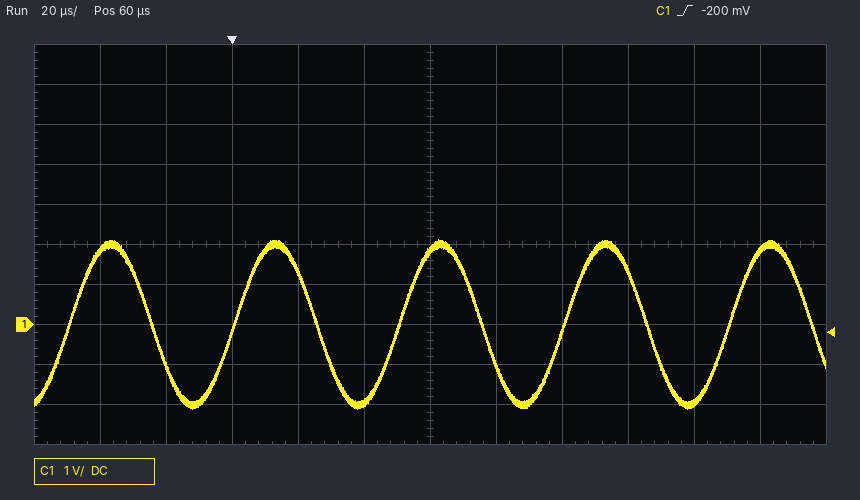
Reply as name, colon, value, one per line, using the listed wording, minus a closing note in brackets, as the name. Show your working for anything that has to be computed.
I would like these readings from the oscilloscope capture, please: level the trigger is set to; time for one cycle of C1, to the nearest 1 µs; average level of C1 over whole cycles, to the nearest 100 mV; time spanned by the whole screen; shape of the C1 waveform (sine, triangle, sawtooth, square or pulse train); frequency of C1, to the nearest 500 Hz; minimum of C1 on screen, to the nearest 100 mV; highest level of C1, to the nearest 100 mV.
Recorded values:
level the trigger is set to: -200 mV
time for one cycle of C1, to the nearest 1 µs: 50 µs
average level of C1 over whole cycles, to the nearest 100 mV: (2.1 V + (-2.1 V)) / 2 ≈ 0.0 V
time spanned by the whole screen: 240 µs
shape of the C1 waveform: sine
frequency of C1, to the nearest 500 Hz: 1 / 50 µs ≈ 20.0 kHz
minimum of C1 on screen, to the nearest 100 mV: -2.1 V
highest level of C1, to the nearest 100 mV: 2.1 V
